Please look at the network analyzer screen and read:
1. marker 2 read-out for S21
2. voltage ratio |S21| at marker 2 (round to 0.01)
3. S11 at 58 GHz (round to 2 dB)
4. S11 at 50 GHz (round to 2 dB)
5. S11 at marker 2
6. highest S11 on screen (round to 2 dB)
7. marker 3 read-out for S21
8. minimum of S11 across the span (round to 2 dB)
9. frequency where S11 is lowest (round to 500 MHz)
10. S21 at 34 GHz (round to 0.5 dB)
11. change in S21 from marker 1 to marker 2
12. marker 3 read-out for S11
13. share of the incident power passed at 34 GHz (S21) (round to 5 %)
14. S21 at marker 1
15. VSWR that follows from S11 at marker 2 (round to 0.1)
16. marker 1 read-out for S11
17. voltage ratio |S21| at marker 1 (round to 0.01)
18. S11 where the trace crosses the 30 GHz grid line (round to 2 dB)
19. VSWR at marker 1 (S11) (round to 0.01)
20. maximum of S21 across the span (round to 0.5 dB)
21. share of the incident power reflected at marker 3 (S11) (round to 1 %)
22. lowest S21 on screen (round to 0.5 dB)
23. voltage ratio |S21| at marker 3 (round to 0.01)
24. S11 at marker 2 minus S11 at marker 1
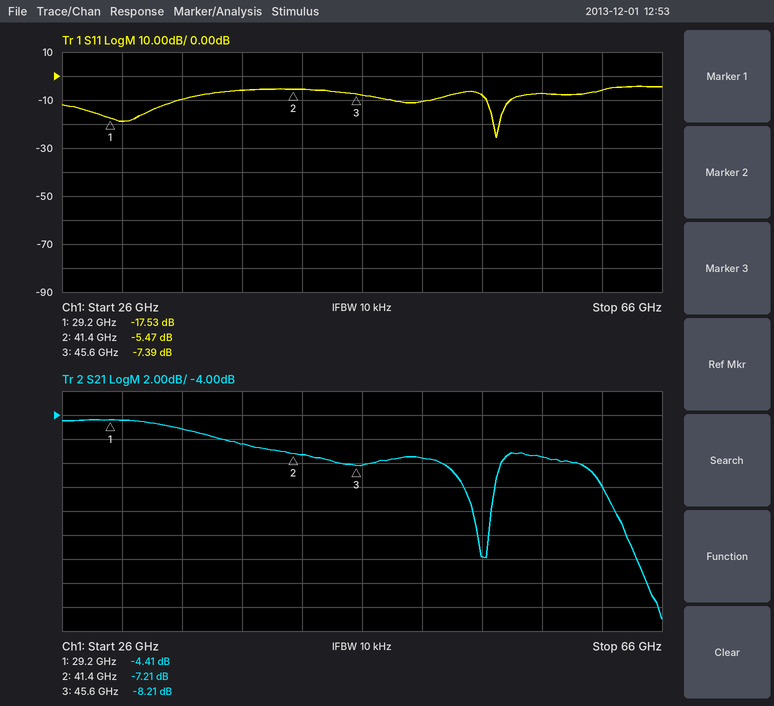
-7.21 dB
0.44
-8 dB
-10 dB
-5.47 dB
-4 dB
-8.21 dB
-26 dB
55.0 GHz
-5.0 dB
-2.80 dB
-7.39 dB
30 %
-4.41 dB
3.3
-17.53 dB
0.60
-18 dB
1.31
-4.5 dB
18 %
-21.0 dB
0.39
12.06 dB
